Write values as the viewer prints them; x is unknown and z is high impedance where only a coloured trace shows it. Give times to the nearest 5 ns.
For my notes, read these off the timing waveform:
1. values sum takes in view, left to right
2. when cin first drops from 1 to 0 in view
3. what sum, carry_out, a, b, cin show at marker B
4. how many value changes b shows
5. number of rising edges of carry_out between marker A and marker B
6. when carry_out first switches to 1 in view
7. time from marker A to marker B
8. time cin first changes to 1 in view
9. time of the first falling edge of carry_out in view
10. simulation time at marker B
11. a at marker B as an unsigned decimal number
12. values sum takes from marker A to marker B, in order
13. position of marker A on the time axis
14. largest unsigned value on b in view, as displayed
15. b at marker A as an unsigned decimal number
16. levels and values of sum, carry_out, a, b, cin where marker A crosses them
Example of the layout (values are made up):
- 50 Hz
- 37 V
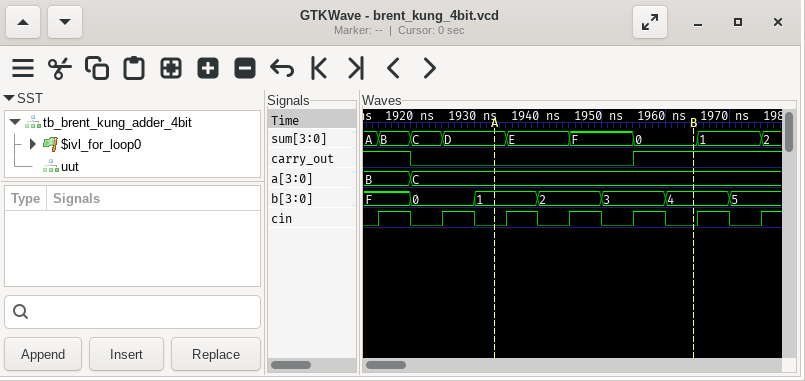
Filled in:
- A, B, C, D, E, F, 0, 1, 2
- 1920 ns
- sum=0, carry_out=1, a=C, b=4, cin=0
- 6
- 1
- 1955 ns
- 30 ns
- 1915 ns
- 1920 ns
- 1965 ns
- 12
- D, E, F, 0
- 1935 ns
- F
- 1
- sum=D, carry_out=0, a=C, b=1, cin=0
